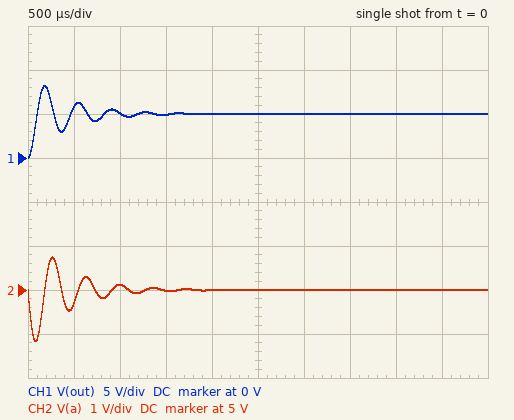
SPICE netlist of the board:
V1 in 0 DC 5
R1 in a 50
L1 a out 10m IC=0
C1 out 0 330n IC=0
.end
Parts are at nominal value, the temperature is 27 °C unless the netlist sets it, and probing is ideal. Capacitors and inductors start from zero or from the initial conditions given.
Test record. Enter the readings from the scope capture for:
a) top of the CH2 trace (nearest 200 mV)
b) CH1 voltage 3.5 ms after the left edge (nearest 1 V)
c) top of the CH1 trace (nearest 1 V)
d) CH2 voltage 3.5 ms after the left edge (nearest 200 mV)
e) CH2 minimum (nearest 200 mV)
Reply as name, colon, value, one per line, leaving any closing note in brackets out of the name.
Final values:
top of the CH2 trace: 5.8 V
CH1 voltage 3.5 ms after the left edge: 5 V
top of the CH1 trace: 8 V
CH2 voltage 3.5 ms after the left edge: 5.0 V
CH2 minimum: 3.8 V
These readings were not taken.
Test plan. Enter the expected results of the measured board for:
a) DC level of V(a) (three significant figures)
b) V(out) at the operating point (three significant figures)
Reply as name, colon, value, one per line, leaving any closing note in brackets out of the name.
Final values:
DC level of V(a): 5.00 V
V(out) at the operating point: 5.00 V
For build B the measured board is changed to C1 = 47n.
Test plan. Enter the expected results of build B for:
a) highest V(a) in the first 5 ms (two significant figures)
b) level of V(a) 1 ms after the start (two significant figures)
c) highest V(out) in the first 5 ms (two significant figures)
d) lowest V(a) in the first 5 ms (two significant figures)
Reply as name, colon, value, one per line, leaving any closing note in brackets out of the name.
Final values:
highest V(a) in the first 5 ms: 5.4 V
level of V(a) 1 ms after the start: 5.0 V
highest V(out) in the first 5 ms: 9.2 V
lowest V(a) in the first 5 ms: 4.5 V
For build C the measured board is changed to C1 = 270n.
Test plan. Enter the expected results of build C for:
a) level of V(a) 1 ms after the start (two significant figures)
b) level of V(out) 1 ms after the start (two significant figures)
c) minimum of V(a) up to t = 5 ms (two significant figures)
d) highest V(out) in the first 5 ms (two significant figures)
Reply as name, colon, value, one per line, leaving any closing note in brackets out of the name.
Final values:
level of V(a) 1 ms after the start: 5.0 V
level of V(out) 1 ms after the start: 4.6 V
minimum of V(a) up to t = 5 ms: 3.9 V
highest V(out) in the first 5 ms: 8.3 V
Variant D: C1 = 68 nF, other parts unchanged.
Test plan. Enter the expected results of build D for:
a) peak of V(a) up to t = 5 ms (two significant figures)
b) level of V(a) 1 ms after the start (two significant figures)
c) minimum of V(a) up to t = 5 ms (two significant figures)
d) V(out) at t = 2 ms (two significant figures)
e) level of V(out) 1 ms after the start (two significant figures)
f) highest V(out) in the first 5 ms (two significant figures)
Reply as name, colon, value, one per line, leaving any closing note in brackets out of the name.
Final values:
peak of V(a) up to t = 5 ms: 5.5 V
level of V(a) 1 ms after the start: 5.0 V
minimum of V(a) up to t = 5 ms: 4.4 V
V(out) at t = 2 ms: 5.0 V
level of V(out) 1 ms after the start: 4.6 V
highest V(out) in the first 5 ms: 9.1 V
